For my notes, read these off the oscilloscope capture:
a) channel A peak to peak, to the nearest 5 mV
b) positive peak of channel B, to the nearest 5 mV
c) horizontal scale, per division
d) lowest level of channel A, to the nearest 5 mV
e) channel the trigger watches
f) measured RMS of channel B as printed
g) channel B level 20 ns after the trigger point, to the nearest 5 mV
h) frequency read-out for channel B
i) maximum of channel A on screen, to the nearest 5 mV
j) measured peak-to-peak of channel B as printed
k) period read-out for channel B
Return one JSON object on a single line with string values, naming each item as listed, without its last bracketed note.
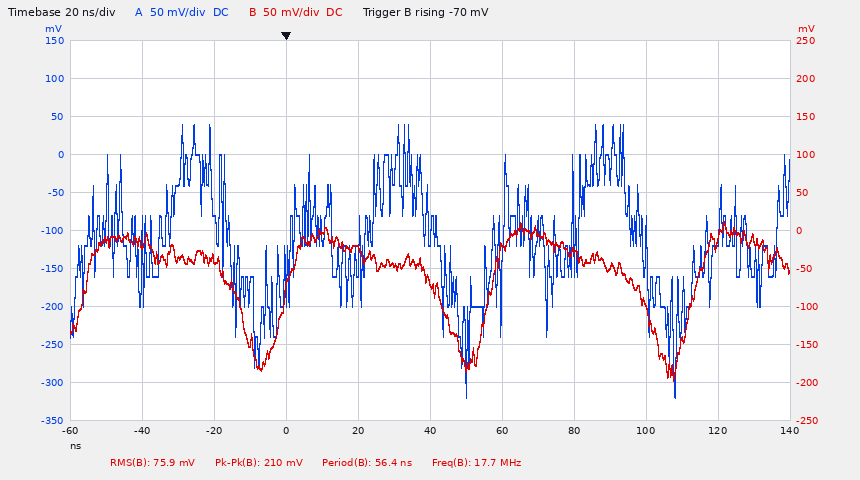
{"channel A peak to peak, to the nearest 5 mV": "360 mV", "positive peak of channel B, to the nearest 5 mV": "10 mV", "horizontal scale, per division": "20 ns", "lowest level of channel A, to the nearest 5 mV": "-320 mV", "channel the trigger watches": "channel B", "measured RMS of channel B as printed": "75.9 mV", "channel B level 20 ns after the trigger point, to the nearest 5 mV": "-25 mV", "frequency read-out for channel B": "17.7 MHz", "maximum of channel A on screen, to the nearest 5 mV": "40 mV", "measured peak-to-peak of channel B as printed": "210 mV", "period read-out for channel B": "56.4 ns"}
